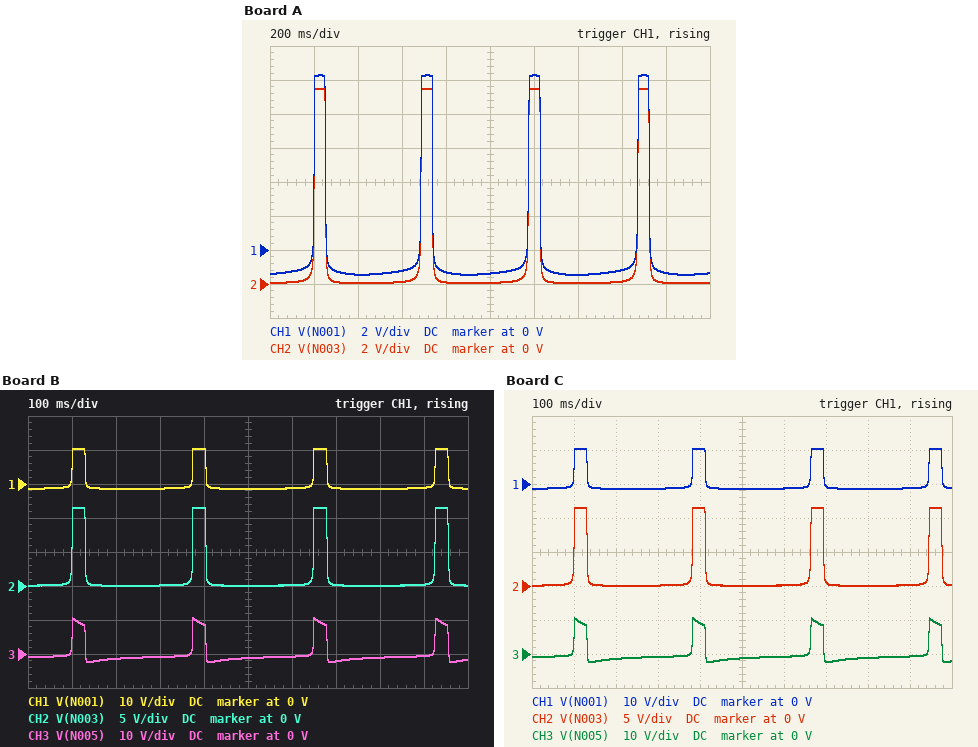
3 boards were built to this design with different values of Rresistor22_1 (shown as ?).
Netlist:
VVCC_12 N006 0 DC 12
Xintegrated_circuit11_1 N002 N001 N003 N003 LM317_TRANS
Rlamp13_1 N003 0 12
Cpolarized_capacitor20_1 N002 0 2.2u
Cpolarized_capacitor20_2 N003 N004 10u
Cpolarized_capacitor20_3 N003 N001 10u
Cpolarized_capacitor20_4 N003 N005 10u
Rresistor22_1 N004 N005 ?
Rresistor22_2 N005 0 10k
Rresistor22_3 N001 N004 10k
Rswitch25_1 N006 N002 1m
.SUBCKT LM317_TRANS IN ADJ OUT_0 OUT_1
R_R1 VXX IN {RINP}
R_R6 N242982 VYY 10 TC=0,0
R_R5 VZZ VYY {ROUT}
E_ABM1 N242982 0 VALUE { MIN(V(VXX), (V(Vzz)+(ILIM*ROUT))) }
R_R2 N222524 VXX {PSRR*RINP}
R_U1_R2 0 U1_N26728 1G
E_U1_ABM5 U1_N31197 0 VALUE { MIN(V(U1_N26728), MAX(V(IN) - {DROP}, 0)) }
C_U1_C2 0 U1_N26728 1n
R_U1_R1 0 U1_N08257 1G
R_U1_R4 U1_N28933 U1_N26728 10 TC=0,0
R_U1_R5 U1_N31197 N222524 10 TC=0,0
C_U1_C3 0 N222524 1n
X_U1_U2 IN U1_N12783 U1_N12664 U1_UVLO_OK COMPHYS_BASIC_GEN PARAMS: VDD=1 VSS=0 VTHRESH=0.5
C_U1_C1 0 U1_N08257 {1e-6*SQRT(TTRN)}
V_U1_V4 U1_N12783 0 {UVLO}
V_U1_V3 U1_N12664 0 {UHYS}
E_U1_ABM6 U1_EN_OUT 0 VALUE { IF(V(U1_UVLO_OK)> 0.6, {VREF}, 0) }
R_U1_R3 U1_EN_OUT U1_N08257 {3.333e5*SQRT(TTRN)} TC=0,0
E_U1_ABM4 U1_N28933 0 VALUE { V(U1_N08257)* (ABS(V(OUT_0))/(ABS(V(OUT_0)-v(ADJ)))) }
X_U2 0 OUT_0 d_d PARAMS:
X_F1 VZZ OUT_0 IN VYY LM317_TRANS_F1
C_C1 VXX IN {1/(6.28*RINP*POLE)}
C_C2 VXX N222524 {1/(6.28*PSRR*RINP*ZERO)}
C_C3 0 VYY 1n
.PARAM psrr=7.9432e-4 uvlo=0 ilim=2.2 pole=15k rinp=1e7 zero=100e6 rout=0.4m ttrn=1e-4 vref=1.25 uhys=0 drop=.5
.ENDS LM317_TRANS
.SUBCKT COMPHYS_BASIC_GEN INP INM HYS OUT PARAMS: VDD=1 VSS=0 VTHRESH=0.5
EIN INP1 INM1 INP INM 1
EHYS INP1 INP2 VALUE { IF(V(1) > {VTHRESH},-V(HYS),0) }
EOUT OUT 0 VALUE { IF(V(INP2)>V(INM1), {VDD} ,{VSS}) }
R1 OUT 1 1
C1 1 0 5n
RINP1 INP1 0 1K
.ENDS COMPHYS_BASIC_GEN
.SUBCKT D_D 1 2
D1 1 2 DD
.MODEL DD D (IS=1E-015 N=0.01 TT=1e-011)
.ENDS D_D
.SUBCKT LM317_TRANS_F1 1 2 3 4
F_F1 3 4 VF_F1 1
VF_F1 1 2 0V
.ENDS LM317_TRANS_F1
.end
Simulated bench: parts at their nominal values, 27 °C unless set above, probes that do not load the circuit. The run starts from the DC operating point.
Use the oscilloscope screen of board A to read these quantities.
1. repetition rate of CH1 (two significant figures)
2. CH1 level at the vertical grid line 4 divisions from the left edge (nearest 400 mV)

2.0 Hz
-1.2 V
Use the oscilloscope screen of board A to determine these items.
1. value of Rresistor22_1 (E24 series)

33 kΩ
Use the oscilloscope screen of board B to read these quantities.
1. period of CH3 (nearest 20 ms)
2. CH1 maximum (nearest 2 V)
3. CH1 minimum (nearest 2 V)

280 ms
10 V
-2 V
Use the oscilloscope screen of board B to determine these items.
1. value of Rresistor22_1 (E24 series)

4.7 kΩ
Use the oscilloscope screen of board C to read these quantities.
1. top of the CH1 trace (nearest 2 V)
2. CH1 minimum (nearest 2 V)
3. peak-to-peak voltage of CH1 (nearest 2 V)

10 V
-2 V
12 V
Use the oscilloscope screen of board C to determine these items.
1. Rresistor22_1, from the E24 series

5.1 kΩ
